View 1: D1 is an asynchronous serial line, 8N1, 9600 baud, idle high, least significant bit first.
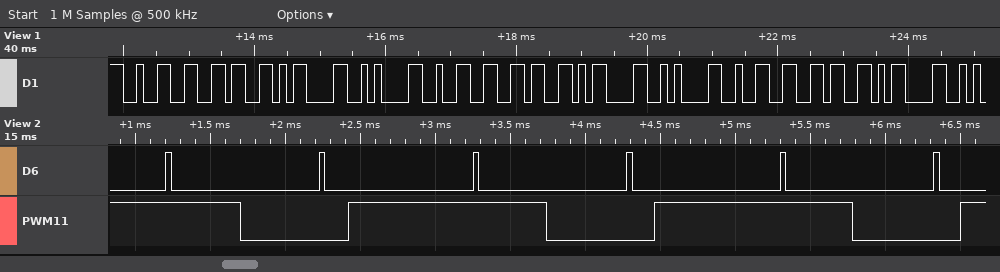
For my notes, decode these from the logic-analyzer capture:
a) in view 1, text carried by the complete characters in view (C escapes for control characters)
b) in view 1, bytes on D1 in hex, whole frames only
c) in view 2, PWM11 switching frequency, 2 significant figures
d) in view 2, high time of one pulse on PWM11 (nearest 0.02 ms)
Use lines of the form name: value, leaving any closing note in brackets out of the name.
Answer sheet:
in view 1, text carried by the complete characters in view: "26\r\n26\r\n26\r"
in view 1, bytes on D1 in hex, whole frames only: 0x32 0x36 0x0D 0x0A 0x32 0x36 0x0D 0x0A 0x32 0x36 0x0D
in view 2, PWM11 switching frequency, 2 significant figures: 490 Hz
in view 2, high time of one pulse on PWM11: 1.32 ms
